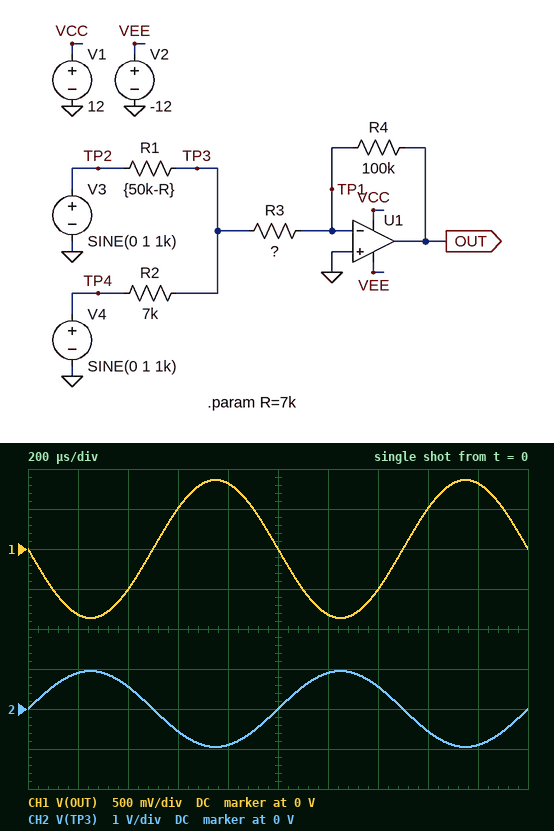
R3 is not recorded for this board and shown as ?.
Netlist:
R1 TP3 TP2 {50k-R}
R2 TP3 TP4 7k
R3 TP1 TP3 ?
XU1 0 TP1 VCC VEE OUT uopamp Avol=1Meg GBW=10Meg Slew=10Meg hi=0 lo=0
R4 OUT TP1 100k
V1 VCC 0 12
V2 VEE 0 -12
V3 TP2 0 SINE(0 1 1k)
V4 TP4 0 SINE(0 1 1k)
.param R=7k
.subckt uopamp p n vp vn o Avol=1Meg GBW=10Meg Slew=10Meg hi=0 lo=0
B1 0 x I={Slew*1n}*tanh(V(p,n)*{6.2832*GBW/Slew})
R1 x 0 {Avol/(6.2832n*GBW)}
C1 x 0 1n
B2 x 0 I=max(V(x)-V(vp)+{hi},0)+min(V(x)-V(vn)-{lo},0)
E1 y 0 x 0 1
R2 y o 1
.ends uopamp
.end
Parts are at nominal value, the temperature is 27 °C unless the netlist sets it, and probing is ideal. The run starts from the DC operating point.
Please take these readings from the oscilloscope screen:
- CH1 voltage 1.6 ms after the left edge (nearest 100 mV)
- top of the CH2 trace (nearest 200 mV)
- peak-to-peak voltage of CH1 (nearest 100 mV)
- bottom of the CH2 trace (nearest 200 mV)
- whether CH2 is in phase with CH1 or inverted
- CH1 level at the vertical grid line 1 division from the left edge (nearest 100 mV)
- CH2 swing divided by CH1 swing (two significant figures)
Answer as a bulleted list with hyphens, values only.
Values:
- 500 mV
- 1.0 V
- 1.7 V
- -1.0 V
- inverted
- -800 mV
- 1.1
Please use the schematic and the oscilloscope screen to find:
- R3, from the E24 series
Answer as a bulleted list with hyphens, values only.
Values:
- 110 kΩ
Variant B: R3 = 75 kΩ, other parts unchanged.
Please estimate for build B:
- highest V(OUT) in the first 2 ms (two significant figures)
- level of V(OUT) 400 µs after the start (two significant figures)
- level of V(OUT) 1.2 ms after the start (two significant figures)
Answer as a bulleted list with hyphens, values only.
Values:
- 1.2 V
- -730 mV
- -1.2 V
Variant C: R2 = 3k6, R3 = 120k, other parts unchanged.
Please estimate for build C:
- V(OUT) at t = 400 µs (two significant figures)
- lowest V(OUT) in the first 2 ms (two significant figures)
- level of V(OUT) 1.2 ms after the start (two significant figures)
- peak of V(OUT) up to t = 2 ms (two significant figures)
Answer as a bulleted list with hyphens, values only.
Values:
- -480 mV
- -810 mV
- -770 mV
- 810 mV
